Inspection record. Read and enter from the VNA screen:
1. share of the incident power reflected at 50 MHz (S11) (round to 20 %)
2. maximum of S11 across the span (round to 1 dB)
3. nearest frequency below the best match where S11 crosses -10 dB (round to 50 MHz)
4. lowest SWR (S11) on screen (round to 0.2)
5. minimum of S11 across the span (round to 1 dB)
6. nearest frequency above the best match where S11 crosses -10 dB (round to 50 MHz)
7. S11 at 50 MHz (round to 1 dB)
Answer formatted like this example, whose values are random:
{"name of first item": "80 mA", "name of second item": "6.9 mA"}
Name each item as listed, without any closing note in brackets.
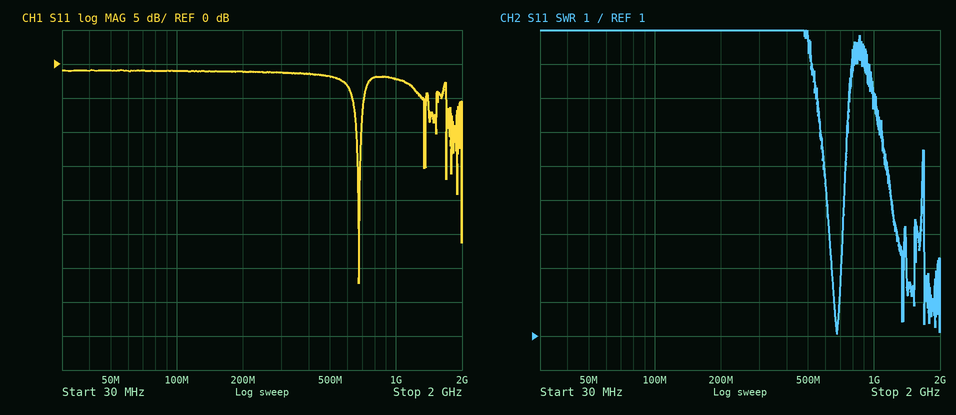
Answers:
{"share of the incident power reflected at 50 MHz (S11)": "80 %", "maximum of S11 across the span": "-1 dB", "nearest frequency below the best match where S11 crosses -10 dB": "650 MHz", "lowest SWR (S11) on screen": "1.0", "minimum of S11 across the span": "-32 dB", "nearest frequency above the best match where S11 crosses -10 dB": "700 MHz", "S11 at 50 MHz": "-1 dB"}
